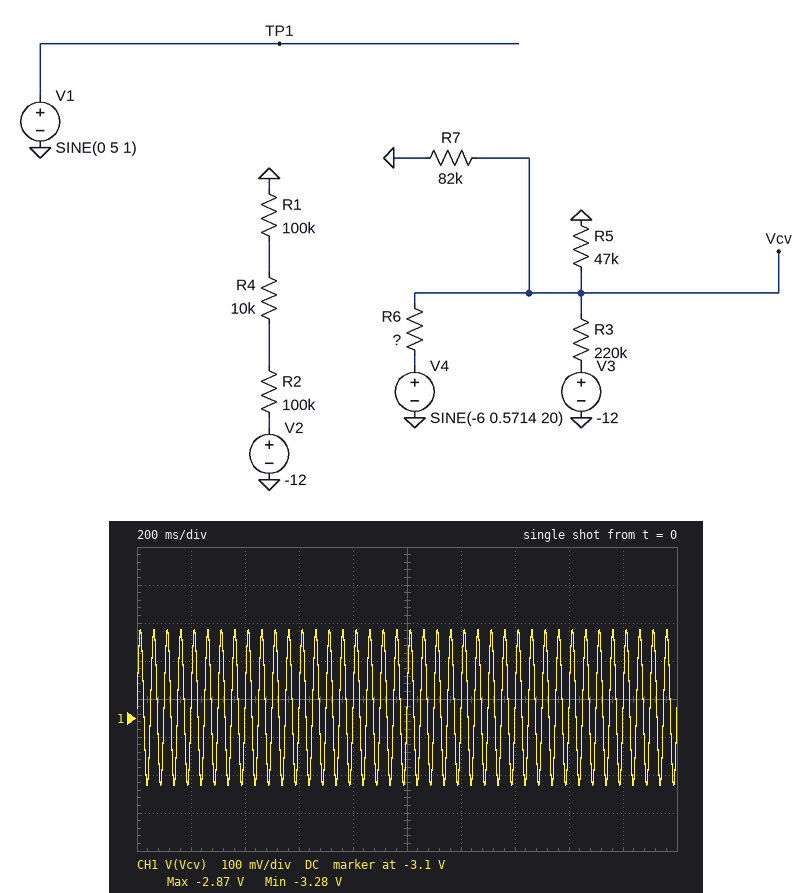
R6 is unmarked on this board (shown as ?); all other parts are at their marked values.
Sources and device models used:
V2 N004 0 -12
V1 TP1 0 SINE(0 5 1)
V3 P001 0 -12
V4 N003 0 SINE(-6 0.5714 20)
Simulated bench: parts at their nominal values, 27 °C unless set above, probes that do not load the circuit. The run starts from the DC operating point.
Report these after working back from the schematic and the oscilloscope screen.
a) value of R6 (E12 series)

47 kΩ
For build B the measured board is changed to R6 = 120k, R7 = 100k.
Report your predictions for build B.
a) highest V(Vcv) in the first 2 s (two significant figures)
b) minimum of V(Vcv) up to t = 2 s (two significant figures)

-2.3 V
-2.5 V
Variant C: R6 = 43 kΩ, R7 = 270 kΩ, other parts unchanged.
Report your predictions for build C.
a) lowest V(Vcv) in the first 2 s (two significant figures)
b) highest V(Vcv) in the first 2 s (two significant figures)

-3.9 V
-3.4 V
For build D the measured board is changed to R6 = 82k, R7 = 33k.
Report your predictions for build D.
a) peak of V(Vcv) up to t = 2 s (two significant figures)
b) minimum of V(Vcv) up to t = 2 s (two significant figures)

-1.8 V
-2.0 V
